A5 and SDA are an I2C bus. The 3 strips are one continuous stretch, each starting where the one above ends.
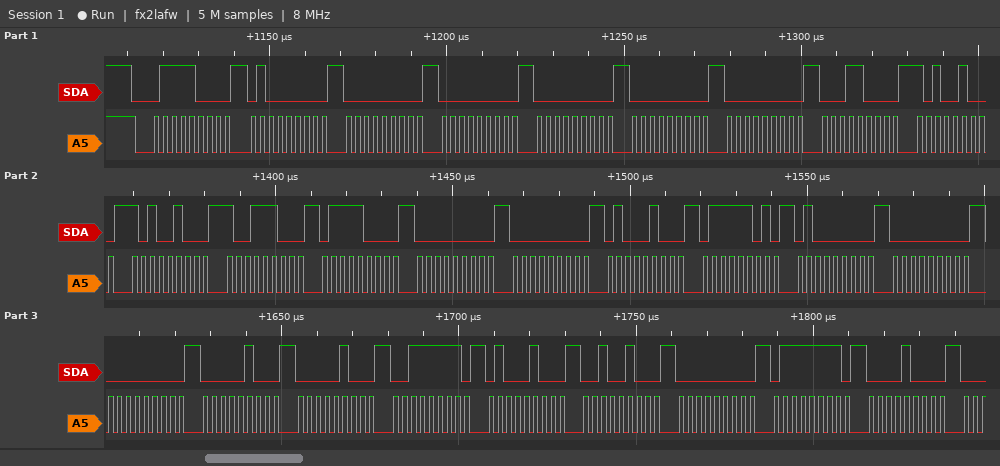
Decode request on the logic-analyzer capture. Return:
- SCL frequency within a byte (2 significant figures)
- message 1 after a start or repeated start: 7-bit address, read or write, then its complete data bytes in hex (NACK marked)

400 kHz
0x3C write: 40 00 00 00 00 00 18 A4 A4 9C 78 00 00 44 7D 40 00 00 04 04 3F 44 24 00 7F 08
